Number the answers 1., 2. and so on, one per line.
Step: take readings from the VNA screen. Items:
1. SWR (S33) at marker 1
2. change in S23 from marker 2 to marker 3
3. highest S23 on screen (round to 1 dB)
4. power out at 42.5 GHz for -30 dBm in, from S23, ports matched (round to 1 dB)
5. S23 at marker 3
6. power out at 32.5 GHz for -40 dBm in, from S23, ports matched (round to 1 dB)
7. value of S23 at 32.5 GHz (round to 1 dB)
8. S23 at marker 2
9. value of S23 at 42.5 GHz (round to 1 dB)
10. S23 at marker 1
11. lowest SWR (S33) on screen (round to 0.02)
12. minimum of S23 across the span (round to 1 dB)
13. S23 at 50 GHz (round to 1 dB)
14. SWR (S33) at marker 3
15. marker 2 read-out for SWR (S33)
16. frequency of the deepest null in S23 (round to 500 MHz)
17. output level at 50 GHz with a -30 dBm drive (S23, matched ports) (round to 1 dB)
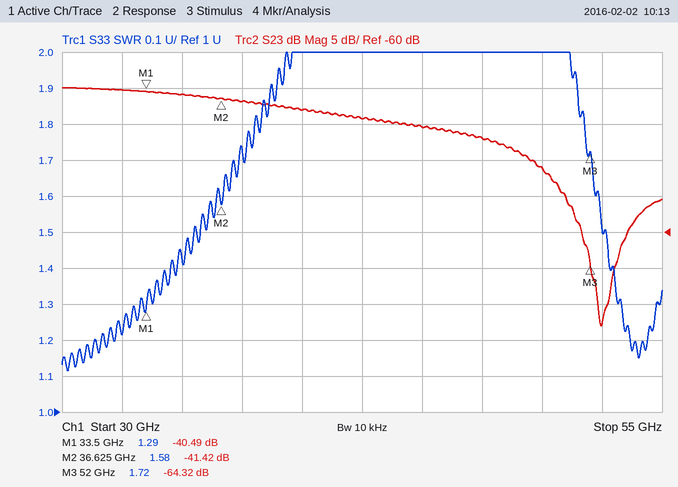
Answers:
1. 1.29
2. -22.90 dB
3. -40 dB
4. -74 dBm
5. -64.32 dB
6. -80 dBm
7. -40 dB
8. -41.42 dB
9. -44 dB
10. -40.49 dB
11. 1.12
12. -73 dB
13. -51 dB
14. 1.72
15. 1.58
16. 52.5 GHz
17. -81 dBm
